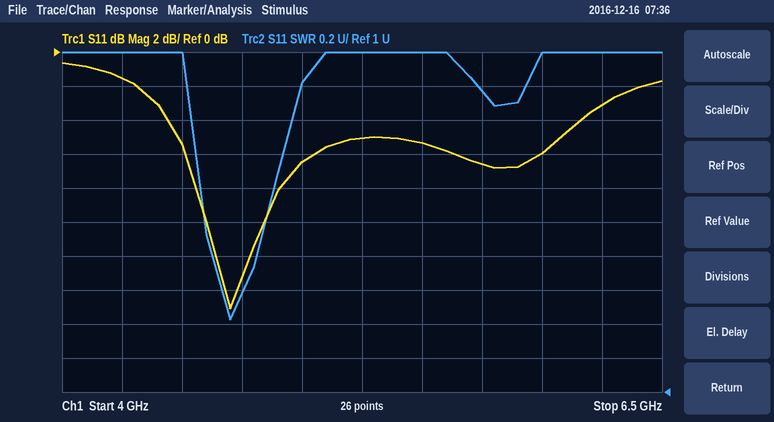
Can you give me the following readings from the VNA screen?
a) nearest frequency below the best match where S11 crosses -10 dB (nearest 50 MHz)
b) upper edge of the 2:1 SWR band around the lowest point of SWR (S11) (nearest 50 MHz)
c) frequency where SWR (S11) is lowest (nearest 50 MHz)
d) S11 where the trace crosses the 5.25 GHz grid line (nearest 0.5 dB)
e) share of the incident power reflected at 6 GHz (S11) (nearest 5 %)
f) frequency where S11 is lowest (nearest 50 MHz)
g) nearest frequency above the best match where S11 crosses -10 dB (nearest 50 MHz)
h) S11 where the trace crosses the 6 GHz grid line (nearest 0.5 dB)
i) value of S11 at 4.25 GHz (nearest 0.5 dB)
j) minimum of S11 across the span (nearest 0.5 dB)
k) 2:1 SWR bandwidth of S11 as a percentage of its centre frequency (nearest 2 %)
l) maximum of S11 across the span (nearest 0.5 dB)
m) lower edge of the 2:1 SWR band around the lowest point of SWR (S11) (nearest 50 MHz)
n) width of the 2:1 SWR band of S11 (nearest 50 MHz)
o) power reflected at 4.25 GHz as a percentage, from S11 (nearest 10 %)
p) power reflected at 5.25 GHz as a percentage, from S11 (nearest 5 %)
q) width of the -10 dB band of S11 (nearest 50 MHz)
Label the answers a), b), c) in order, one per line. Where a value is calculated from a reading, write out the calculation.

a) 4.60 GHz
b) 4.85 GHz
c) 4.70 GHz
d) -5.0 dB
e) 10^(-6/10) ≈ 25 %
f) 4.70 GHz
g) 4.85 GHz
h) -6.0 dB
i) -1.5 dB
j) -15.0 dB
k) 250 MHz / 4.725 GHz ≈ 5.29 %, so 6 % to the nearest 2 %
l) -0.5 dB
m) 4.60 GHz
n) 4.85 GHz − 4.60 GHz = 250 MHz
o) 10^(-1.5/10) ≈ 70.8 %, so 70 % to the nearest 10 %
p) 10^(-5/10) ≈ 31.6 %, so 30 % to the nearest 5 %
q) 4.85 GHz − 4.60 GHz = 250 MHz
